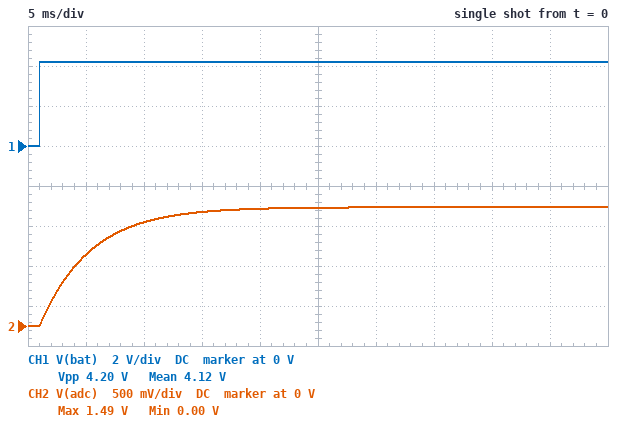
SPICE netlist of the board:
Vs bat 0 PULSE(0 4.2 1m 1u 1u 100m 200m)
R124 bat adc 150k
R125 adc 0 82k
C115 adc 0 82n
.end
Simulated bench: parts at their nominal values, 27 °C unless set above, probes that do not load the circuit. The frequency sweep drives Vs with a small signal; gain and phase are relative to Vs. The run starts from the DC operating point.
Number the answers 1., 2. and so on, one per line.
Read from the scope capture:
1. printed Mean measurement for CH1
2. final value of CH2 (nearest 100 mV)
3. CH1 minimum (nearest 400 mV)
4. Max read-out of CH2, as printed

1. 4.12 V
2. 1.5 V
3. 0 V
4. 1.49 V
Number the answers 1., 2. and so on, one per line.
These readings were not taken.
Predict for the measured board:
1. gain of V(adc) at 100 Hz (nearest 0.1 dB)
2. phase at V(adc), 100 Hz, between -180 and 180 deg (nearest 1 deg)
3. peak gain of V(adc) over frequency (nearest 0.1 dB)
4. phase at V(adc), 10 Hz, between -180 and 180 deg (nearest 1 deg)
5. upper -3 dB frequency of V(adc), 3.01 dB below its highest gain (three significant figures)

1. -18.3 dB
2. -70 deg
3. -9.0 dB
4. -15 deg
5. 36.6 Hz
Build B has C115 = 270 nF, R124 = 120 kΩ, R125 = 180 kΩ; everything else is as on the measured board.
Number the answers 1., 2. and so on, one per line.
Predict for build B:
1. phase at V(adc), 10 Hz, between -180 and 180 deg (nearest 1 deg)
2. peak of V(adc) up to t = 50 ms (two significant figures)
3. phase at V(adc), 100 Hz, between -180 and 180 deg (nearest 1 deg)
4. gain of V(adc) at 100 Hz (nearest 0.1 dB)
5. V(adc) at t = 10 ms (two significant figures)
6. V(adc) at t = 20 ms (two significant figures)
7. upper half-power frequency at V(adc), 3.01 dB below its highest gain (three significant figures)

1. -51 deg
2. 2.3 V
3. -85 deg
4. -26.2 dB
5. 930 mV
6. 1.6 V
7. 8.19 Hz
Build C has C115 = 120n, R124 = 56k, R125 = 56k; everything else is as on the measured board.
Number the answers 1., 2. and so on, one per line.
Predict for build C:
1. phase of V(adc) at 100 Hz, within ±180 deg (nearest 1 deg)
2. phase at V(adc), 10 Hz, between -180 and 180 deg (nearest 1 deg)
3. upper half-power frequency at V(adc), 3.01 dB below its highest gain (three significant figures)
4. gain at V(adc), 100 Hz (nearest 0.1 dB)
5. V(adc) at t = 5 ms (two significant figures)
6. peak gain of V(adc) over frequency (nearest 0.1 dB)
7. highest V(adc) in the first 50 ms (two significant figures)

1. -65 deg
2. -12 deg
3. 47.4 Hz
4. -13.4 dB
5. 1.5 V
6. -6.0 dB
7. 2.1 V
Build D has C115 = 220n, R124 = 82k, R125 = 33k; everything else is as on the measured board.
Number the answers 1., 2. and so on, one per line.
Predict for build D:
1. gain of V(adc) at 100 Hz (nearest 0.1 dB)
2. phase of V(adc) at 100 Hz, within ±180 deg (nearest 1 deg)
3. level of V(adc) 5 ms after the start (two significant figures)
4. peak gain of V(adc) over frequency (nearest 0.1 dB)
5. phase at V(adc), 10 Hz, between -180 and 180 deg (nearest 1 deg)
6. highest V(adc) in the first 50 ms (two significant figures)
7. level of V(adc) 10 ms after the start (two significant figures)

1. -21.5 dB
2. -73 deg
3. 650 mV
4. -10.8 dB
5. -18 deg
6. 1.2 V
7. 990 mV
